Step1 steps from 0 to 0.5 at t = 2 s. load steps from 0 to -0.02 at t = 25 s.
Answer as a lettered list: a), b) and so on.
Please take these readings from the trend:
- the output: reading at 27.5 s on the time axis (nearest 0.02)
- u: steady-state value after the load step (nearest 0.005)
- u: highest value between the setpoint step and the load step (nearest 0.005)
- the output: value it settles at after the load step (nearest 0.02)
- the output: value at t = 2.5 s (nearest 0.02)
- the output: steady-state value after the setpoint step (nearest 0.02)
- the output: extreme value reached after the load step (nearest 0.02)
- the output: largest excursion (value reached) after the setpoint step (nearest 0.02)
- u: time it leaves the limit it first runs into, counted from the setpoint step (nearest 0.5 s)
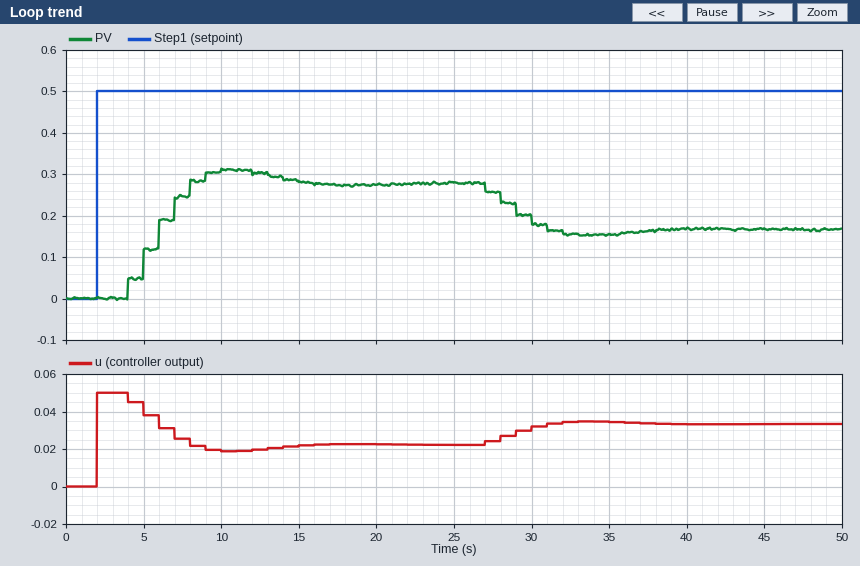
a) 0.26
b) 0.035
c) 0.050
d) 0.16
e) 0.00
f) 0.28
g) 0.16
h) 0.32
i) 2.0 s
